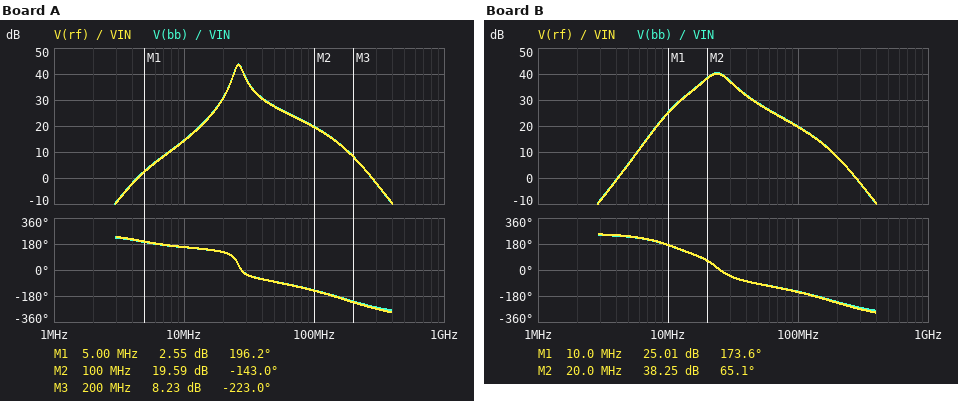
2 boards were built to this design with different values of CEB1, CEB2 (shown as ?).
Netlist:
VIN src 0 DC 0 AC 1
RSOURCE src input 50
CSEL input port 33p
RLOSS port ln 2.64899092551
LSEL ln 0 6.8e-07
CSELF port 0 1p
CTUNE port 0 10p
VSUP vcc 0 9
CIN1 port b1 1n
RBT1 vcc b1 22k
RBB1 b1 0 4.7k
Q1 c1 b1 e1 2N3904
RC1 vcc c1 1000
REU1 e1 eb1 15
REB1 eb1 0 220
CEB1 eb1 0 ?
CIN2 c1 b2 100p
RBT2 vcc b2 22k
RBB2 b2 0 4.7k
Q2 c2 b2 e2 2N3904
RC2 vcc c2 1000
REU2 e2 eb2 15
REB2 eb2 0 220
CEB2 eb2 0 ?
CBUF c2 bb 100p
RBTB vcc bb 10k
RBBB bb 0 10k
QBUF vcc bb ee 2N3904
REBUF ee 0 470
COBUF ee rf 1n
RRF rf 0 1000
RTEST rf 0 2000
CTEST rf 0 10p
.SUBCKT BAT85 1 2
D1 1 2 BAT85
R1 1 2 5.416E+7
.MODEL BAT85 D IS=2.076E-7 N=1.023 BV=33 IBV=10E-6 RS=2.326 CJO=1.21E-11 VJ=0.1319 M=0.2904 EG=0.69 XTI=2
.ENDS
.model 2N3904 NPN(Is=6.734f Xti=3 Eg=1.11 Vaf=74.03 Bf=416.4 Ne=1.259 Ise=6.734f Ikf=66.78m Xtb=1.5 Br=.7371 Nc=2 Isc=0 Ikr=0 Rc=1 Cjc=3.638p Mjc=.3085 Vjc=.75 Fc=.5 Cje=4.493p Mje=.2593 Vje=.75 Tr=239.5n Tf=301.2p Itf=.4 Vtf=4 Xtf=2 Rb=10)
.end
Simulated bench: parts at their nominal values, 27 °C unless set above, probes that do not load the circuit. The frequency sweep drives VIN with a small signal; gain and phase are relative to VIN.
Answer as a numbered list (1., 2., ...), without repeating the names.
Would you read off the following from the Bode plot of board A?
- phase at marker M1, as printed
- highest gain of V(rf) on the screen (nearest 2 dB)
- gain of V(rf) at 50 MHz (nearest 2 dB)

1. 196.2 deg
2. 44 dB
3. 28 dB
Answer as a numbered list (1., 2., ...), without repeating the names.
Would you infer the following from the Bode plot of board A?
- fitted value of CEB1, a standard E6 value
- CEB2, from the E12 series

1. 150 pF
2. 820 pF
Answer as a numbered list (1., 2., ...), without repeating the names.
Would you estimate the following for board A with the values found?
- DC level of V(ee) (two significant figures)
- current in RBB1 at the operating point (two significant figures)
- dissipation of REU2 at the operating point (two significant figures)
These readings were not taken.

1. 3.6 V
2. 320 µA
3. 180 µW
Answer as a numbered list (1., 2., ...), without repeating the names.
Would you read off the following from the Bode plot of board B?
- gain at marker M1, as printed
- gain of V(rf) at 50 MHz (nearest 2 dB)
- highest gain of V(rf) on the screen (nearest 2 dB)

1. 25.01 dB
2. 28 dB
3. 40 dB
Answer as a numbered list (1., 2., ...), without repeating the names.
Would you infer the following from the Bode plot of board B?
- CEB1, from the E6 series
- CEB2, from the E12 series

1. 1 nF
2. 150 pF
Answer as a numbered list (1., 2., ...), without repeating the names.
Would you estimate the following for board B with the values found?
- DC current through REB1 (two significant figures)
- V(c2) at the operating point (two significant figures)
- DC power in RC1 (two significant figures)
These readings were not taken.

1. 3.4 mA
2. 5.6 V
3. 12 mW
